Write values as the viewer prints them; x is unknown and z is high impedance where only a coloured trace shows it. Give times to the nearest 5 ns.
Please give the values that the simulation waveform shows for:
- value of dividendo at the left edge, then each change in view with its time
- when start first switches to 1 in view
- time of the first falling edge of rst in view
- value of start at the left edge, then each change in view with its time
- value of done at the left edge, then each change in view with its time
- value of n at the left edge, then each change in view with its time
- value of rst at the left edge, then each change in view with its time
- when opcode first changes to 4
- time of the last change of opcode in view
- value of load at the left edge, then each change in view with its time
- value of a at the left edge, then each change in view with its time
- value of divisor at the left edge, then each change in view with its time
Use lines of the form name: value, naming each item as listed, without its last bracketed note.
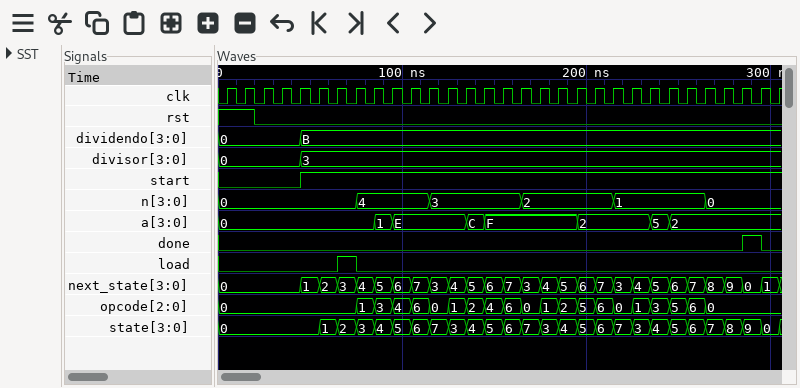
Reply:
value of dividendo at the left edge, then each change in view with its time: 0, B at 45 ns
when start first switches to 1 in view: 45 ns
time of the first falling edge of rst in view: 20 ns
value of start at the left edge, then each change in view with its time: 0, 1 at 45 ns
value of done at the left edge, then each change in view with its time: 0, 1 at 285 ns, 0 at 295 ns
value of n at the left edge, then each change in view with its time: 0, 4 at 75 ns, 3 at 115 ns, 2 at 165 ns, 1 at 215 ns, 0 at 265 ns
value of rst at the left edge, then each change in view with its time: 1, 0 at 20 ns
when opcode first changes to 4: 95 ns
time of the last change of opcode in view: 265 ns
value of load at the left edge, then each change in view with its time: 0, 1 at 65 ns, 0 at 75 ns
value of a at the left edge, then each change in view with its time: 0, 1 at 85 ns, E at 95 ns, C at 135 ns, F at 145 ns, 2 at 195 ns, 5 at 235 ns, 2 at 245 ns
value of divisor at the left edge, then each change in view with its time: 0, 3 at 45 ns
